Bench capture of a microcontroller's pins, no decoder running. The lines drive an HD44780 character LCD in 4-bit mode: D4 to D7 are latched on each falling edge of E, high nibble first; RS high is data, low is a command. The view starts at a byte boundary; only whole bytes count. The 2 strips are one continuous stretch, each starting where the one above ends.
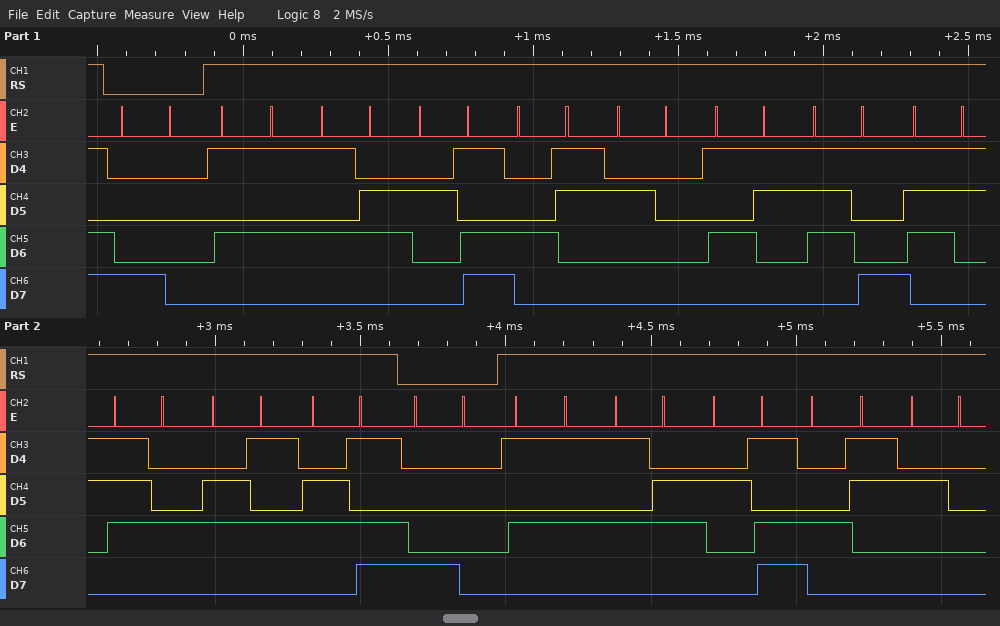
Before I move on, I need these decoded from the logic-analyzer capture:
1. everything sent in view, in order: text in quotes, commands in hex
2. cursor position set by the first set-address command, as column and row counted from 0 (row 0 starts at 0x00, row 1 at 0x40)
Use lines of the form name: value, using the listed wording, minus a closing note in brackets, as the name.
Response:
everything sent in view, in order: text in quotes, commands in hex: 0x80 "UV-C System" 0x80 "UV-C "
cursor position set by the first set-address command, as column and row counted from 0: column 0, row 0
